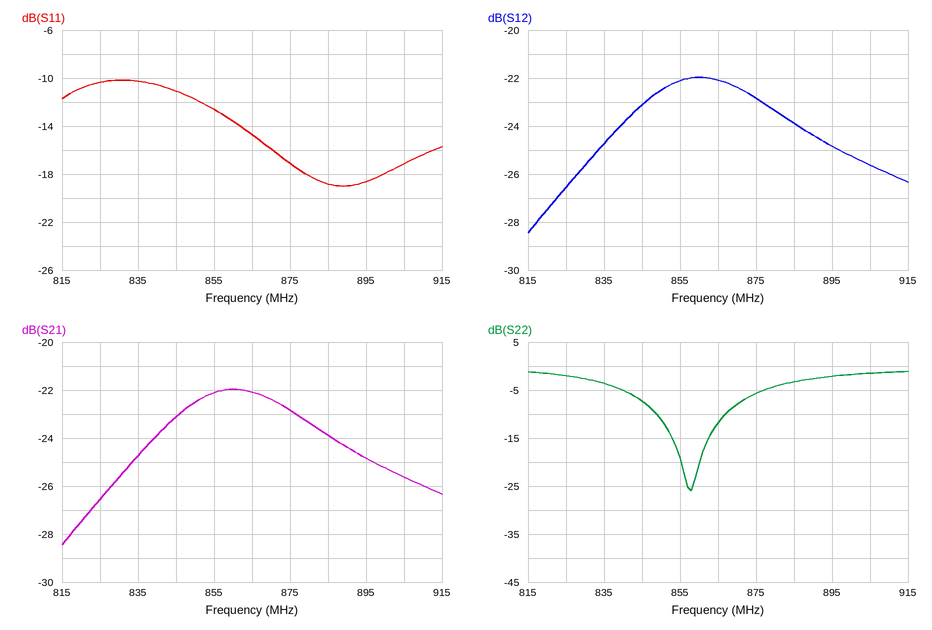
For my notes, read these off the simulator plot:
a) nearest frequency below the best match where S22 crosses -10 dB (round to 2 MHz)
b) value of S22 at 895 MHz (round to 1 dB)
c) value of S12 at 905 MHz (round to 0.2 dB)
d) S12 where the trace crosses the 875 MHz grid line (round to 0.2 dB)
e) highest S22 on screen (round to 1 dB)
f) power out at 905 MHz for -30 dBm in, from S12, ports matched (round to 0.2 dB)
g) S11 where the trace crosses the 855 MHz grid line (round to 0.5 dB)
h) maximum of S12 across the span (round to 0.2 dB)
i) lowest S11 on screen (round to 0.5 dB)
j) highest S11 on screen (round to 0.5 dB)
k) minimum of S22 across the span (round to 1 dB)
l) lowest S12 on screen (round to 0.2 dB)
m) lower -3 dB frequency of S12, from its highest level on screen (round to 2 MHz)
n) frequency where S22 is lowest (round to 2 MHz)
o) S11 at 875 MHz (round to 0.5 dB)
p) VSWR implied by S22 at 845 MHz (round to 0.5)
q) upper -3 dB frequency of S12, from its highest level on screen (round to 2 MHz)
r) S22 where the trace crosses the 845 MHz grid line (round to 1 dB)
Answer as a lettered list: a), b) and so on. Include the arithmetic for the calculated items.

a) 848 MHz
b) -2 dB
c) -25.6 dB
d) -22.8 dB
e) -1 dB
f) -30 dBm + (-25.6 dB) = -55.6 dBm
g) -12.5 dB
h) -22.0 dB
i) -19.0 dB
j) -10.0 dB
k) -26 dB
l) -28.4 dB
m) 834 MHz
n) 858 MHz
o) -17.0 dB
p) |Γ| = 10^(-7/20) = 0.4467; VSWR = (1 + 0.4467)/(1 − 0.4467) ≈ 2.61, so 2.5 to the nearest 0.5
q) 896 MHz
r) -7 dB
